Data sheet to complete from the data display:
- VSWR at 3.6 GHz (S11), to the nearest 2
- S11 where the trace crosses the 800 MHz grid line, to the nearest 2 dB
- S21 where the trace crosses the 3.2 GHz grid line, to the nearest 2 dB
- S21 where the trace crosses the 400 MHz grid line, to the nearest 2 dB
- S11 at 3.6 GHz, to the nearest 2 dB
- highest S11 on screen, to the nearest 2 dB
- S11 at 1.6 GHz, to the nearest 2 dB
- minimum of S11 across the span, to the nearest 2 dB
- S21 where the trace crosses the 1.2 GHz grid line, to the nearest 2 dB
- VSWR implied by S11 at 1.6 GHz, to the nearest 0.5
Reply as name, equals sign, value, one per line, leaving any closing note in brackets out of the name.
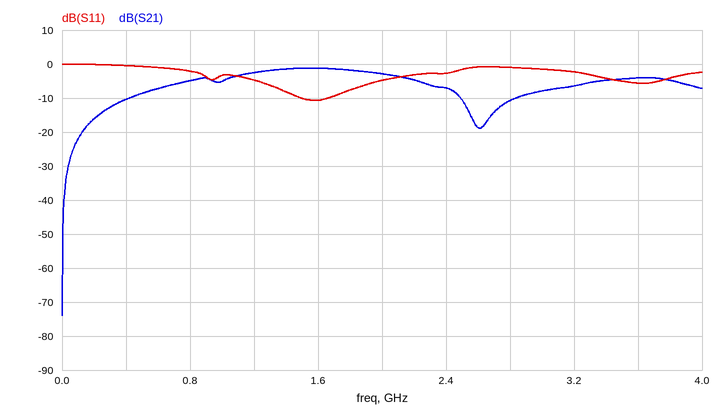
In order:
VSWR at 3.6 GHz (S11), to the nearest 2 = 4
S11 where the trace crosses the 800 MHz grid line, to the nearest 2 dB = -2 dB
S21 where the trace crosses the 3.2 GHz grid line, to the nearest 2 dB = -6 dB
S21 where the trace crosses the 400 MHz grid line, to the nearest 2 dB = -10 dB
S11 at 3.6 GHz, to the nearest 2 dB = -6 dB
highest S11 on screen, to the nearest 2 dB = 0 dB
S11 at 1.6 GHz, to the nearest 2 dB = -10 dB
minimum of S11 across the span, to the nearest 2 dB = -10 dB
S21 where the trace crosses the 1.2 GHz grid line, to the nearest 2 dB = -2 dB
VSWR implied by S11 at 1.6 GHz, to the nearest 0.5 = 2.0
